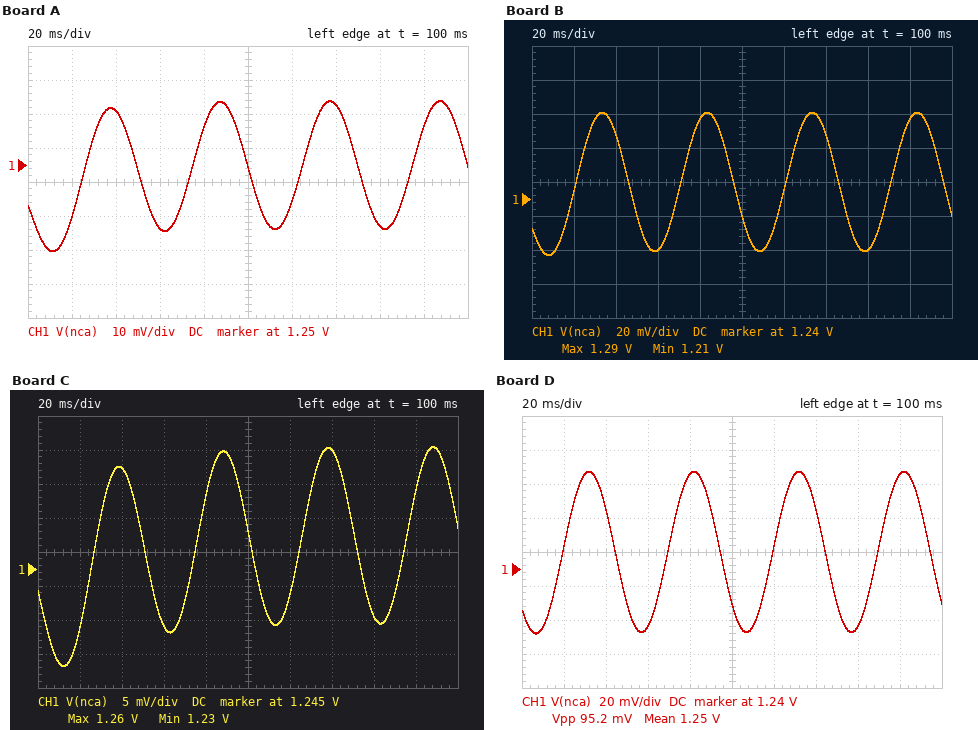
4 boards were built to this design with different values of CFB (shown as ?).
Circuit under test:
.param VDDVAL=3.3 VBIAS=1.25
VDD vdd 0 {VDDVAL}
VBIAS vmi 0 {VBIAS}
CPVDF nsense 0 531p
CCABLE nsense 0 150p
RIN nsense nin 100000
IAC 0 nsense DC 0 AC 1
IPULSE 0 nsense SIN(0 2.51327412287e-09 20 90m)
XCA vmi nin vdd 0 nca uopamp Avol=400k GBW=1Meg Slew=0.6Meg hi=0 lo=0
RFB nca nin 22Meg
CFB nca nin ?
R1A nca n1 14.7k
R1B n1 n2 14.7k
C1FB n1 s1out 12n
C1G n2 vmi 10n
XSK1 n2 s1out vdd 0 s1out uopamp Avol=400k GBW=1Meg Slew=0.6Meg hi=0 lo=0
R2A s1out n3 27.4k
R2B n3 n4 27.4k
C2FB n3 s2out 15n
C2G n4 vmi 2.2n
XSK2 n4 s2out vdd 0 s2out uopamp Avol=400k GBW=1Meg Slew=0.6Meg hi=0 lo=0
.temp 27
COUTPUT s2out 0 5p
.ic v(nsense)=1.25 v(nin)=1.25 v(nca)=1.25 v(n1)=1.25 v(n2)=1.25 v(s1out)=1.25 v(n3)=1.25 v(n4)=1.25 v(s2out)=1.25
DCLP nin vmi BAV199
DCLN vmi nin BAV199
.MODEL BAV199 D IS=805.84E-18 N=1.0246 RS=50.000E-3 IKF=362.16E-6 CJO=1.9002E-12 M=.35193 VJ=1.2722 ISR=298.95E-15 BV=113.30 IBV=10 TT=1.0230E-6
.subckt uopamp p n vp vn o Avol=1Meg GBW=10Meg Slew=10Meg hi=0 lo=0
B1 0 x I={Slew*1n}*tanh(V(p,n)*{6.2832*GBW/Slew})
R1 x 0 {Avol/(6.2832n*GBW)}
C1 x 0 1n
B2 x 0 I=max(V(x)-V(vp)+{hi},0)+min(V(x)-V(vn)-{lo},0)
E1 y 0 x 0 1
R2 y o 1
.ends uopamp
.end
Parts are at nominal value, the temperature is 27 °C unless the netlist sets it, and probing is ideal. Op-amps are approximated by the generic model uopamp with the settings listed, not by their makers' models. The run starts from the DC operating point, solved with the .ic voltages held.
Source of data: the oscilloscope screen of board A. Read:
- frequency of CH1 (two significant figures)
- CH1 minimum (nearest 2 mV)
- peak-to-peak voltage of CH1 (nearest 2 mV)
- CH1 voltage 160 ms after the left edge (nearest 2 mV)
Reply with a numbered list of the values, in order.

1. 20 Hz
2. 1.224 V
3. 44 mV
4. 1.232 V
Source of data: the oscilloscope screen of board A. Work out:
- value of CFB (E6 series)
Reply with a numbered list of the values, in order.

1. 1 nF
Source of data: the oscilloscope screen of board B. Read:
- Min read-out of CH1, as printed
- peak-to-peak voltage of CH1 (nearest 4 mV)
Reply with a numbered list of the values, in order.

1. 1.21 V
2. 84 mV
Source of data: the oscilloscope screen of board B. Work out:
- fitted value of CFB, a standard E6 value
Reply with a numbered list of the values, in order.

1. 330 pF
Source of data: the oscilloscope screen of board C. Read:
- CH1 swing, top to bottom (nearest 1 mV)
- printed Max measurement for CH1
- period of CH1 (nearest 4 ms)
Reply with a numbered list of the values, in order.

1. 32 mV
2. 1.26 V
3. 48 ms
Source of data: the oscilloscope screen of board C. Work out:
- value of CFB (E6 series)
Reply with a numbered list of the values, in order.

1. 1.5 nF
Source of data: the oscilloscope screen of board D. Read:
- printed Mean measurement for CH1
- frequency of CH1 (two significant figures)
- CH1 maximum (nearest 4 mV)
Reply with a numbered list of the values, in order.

1. 1.25 V
2. 20 Hz
3. 1.296 V
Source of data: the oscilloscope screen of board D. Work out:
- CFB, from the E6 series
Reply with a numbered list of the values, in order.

1. 220 pF
